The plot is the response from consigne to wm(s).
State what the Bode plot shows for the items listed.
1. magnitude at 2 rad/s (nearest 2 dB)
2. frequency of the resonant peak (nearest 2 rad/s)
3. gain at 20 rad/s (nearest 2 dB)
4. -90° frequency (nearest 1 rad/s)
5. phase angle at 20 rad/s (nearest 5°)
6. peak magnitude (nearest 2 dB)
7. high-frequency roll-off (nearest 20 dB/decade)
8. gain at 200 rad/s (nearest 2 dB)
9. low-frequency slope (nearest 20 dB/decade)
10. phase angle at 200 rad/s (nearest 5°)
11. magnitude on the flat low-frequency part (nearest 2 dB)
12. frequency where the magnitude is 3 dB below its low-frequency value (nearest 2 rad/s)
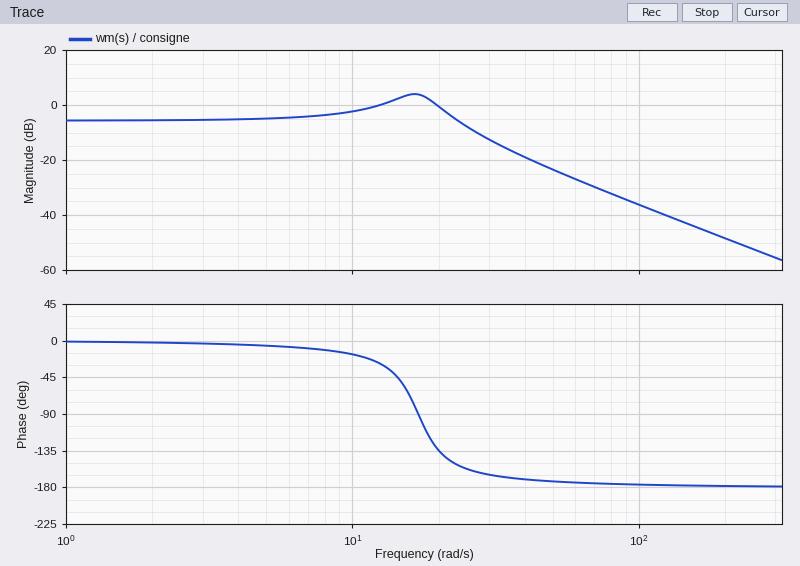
-6 dB
16 rad/s
0 dB
17 rad/s
-135°
4 dB
-40 dB/decade
-48 dB
0 dB/decade
-180°
-6 dB
26 rad/s
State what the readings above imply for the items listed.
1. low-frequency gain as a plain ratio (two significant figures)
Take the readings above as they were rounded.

0.50
